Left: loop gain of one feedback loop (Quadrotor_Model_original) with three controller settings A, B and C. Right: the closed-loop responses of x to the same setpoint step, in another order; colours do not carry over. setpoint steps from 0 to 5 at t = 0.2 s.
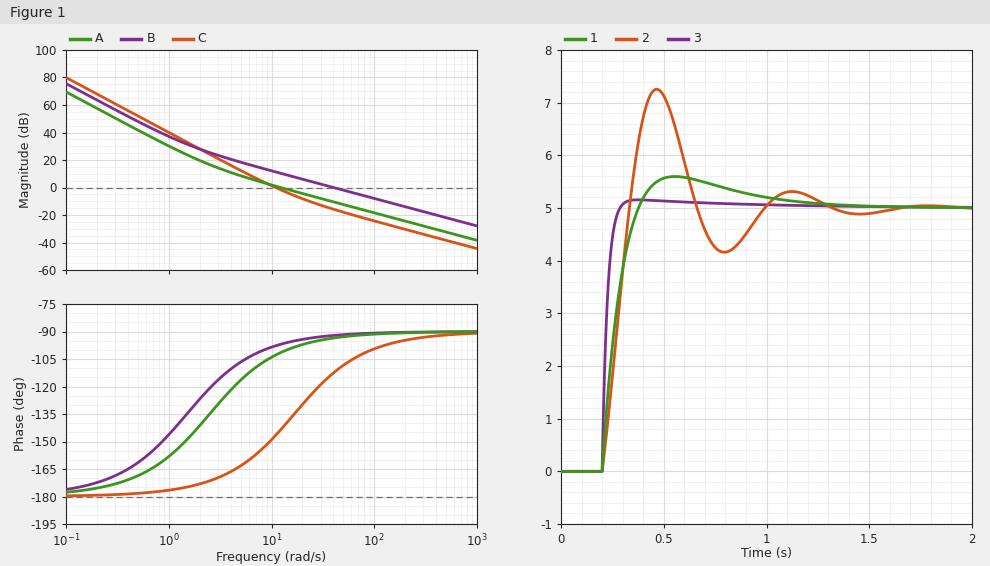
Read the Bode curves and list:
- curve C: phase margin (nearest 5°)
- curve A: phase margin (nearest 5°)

35°
80°
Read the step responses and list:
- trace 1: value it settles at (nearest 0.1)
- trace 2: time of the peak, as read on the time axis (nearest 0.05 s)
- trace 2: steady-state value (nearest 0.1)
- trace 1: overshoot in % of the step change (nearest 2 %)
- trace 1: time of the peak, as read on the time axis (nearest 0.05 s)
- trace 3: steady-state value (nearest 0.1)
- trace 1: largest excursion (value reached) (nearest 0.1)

5.0
0.45 s
5.0
12 %
0.55 s
5.0
5.6
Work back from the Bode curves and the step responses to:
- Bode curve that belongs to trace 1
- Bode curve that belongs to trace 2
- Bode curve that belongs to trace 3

A
C
B
